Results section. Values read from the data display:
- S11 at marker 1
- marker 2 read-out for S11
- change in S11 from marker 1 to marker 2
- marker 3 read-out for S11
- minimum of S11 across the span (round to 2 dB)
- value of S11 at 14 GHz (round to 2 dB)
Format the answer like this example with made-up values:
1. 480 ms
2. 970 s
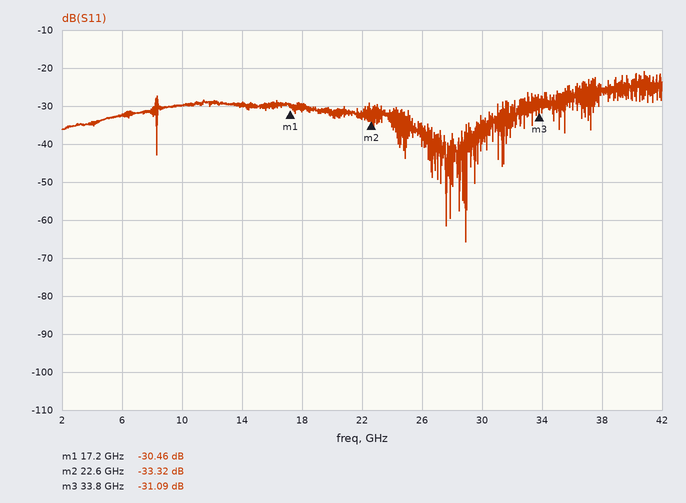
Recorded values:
1. -30.46 dB
2. -33.32 dB
3. -2.86 dB
4. -31.09 dB
5. -66 dB
6. -30 dB
